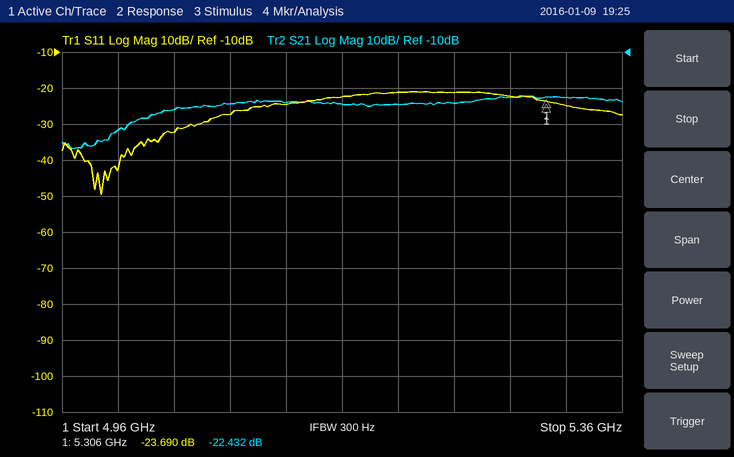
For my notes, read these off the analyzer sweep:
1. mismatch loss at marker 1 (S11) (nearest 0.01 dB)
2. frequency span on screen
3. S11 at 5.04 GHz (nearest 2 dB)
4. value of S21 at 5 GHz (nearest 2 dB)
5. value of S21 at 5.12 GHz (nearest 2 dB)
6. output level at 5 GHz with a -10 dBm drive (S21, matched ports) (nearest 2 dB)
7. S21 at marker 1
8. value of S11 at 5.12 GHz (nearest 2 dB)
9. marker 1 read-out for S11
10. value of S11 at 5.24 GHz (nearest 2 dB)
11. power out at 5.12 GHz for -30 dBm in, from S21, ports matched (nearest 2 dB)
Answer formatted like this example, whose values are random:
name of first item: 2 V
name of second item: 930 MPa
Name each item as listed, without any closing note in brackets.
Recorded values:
mismatch loss at marker 1 (S11): 0.02 dB
frequency span on screen: 400 MHz
S11 at 5.04 GHz: -32 dB
value of S21 at 5 GHz: -32 dB
value of S21 at 5.12 GHz: -24 dB
output level at 5 GHz with a -10 dBm drive (S21, matched ports): -42 dBm
S21 at marker 1: -22.432 dB
value of S11 at 5.12 GHz: -24 dB
marker 1 read-out for S11: -23.690 dB
value of S11 at 5.24 GHz: -22 dB
power out at 5.12 GHz for -30 dBm in, from S21, ports matched: -54 dBm
